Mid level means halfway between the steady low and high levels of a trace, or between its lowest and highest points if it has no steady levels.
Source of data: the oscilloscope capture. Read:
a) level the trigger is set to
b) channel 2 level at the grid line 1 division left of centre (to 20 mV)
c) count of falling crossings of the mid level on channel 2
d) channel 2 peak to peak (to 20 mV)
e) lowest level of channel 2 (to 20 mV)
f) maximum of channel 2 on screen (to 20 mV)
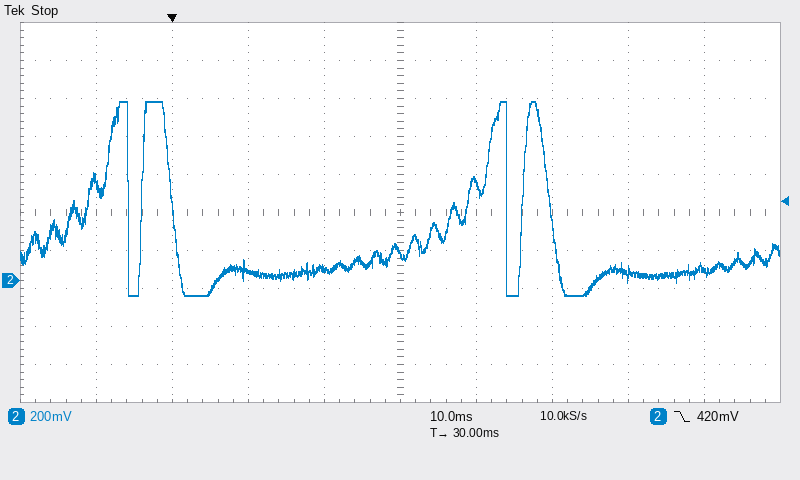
420 mV
60 mV
4
1.02 V
-80 mV
940 mV
